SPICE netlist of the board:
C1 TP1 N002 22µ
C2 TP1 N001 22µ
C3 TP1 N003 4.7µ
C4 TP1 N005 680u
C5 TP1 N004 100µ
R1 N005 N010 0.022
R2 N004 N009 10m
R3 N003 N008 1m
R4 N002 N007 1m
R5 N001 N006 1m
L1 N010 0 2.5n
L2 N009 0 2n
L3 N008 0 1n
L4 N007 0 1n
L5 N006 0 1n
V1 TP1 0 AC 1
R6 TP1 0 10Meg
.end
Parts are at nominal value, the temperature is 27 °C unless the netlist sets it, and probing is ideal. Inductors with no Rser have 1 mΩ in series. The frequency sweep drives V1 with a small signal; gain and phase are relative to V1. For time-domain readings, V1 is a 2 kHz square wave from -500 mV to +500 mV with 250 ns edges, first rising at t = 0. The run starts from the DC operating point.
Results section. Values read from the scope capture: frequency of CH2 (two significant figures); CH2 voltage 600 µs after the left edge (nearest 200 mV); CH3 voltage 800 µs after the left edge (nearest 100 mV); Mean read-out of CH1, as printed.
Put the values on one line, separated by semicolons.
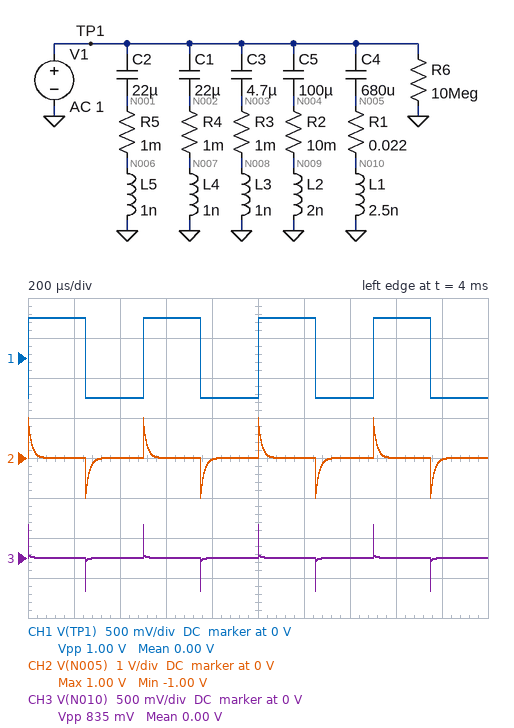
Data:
2.0 kHz; 0 V; 0 V; 0.00 V
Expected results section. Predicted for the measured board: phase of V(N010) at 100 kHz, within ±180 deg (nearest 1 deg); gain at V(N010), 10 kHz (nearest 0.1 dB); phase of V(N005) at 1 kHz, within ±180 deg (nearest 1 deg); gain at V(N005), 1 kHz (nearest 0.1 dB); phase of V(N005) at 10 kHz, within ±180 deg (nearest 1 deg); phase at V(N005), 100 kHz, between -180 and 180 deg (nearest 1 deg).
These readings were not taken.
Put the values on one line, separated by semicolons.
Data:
59 deg; -30.2 dB; 84 deg; -20.2 dB; 46 deg; 6 deg
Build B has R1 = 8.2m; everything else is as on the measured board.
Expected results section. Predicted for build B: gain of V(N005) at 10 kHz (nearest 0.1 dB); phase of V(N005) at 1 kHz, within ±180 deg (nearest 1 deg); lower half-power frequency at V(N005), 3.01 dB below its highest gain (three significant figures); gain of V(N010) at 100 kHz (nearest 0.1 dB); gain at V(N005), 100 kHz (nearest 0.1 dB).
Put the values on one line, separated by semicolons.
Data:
-8.7 dB; 88 deg; 26.0 kHz; -13.9 dB; 0.1 dB
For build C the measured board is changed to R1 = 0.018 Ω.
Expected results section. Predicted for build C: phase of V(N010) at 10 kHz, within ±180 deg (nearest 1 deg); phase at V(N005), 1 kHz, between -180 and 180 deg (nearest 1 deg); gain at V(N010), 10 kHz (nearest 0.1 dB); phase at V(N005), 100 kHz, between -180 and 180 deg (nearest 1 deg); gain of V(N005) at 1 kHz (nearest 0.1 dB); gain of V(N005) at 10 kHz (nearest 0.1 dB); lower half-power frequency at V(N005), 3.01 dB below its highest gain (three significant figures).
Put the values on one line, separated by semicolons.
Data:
60 deg; 85 deg; -29.4 dB; 7 deg; -21.8 dB; -4.0 dB; 12.4 kHz
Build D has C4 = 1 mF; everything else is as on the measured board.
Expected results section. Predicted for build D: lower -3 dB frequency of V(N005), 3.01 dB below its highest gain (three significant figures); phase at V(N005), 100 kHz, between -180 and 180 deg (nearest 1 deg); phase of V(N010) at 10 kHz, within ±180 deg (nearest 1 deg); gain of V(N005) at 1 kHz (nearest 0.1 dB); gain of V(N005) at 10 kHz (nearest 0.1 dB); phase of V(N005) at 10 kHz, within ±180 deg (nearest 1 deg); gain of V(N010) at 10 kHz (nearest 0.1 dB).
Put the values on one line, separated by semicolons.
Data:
6.95 kHz; 4 deg; 43 deg; -16.9 dB; -1.7 dB; 35 deg; -28.8 dB
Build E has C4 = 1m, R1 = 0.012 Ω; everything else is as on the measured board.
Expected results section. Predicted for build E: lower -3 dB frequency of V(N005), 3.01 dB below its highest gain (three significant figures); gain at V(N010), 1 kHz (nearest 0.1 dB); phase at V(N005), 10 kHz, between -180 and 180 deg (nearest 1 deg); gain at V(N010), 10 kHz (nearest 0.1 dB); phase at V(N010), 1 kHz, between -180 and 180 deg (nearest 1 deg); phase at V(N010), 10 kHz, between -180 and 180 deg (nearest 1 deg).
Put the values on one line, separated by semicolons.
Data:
12.4 kHz; -44.1 dB; 51 deg; -26.1 dB; 86 deg; 59 deg
